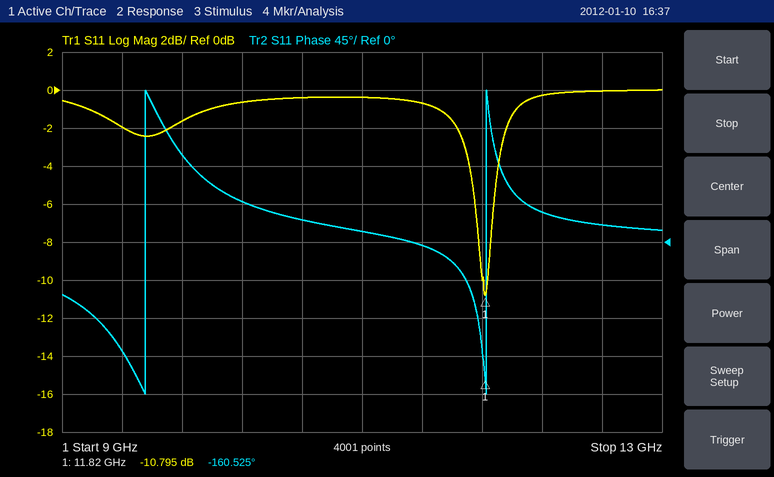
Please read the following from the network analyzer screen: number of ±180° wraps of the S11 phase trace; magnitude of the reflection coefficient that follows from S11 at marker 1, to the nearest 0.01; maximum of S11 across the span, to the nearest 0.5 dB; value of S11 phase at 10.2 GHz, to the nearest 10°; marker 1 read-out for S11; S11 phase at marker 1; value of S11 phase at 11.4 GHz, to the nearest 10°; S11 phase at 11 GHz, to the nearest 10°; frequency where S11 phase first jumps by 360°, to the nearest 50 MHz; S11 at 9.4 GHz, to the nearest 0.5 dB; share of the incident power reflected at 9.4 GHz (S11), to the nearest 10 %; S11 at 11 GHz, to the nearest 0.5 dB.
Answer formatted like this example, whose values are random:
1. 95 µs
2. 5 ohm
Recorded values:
1. 2
2. 0.29
3. 0.0 dB
4. 50°
5. -10.795 dB
6. -160.525°
7. 0°
8. 10°
9. 9.55 GHz
10. -2.0 dB
11. 60 %
12. -0.5 dB
